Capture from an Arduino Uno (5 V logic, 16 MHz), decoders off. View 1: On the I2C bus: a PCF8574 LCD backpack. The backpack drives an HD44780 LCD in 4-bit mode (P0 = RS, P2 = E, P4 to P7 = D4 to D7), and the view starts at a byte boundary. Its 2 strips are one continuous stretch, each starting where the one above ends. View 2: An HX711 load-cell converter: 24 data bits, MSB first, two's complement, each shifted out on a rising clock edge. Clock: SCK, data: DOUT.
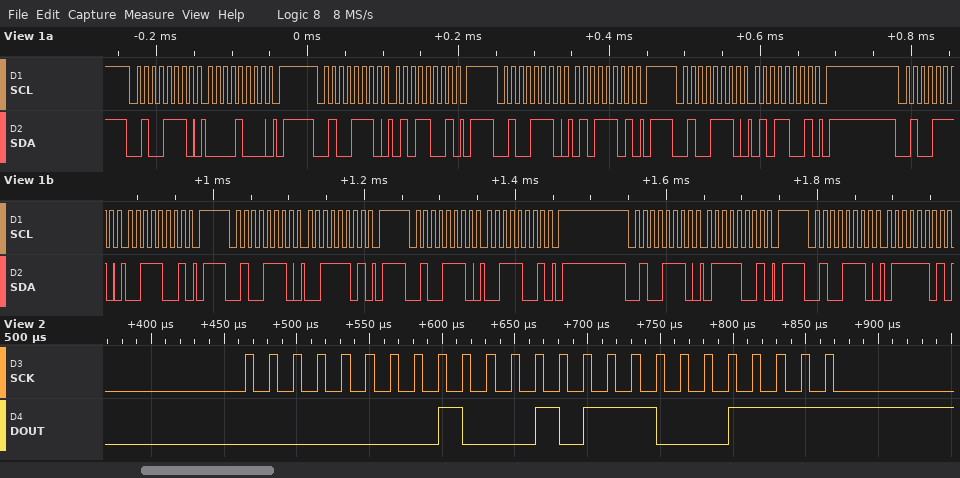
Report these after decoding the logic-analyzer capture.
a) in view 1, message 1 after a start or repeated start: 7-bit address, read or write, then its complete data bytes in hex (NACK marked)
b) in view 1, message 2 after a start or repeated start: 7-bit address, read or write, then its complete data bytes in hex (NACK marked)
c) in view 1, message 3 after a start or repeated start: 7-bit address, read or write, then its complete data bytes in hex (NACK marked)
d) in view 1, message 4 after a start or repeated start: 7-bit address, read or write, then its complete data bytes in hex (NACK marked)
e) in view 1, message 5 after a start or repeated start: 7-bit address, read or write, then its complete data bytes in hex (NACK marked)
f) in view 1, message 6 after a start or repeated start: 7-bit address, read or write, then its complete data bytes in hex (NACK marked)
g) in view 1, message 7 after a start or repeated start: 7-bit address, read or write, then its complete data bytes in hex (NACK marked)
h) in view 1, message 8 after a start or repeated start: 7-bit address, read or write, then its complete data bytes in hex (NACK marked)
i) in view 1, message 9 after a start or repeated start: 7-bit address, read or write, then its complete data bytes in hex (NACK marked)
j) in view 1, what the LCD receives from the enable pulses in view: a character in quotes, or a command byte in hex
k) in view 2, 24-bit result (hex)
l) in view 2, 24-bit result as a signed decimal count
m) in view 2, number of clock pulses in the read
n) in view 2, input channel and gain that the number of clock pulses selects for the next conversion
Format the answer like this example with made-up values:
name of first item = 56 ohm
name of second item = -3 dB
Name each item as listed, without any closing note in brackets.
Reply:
in view 1, message 1 after a start or repeated start: 7-bit address, read or write, then its complete data bytes in hex = 0x27 write: 08
in view 1, message 2 after a start or repeated start: 7-bit address, read or write, then its complete data bytes in hex = 0x27 write: 59
in view 1, message 3 after a start or repeated start: 7-bit address, read or write, then its complete data bytes in hex = 0x27 write: 5D
in view 1, message 4 after a start or repeated start: 7-bit address, read or write, then its complete data bytes in hex = 0x27 write: 59
in view 1, message 5 after a start or repeated start: 7-bit address, read or write, then its complete data bytes in hex = 0x27 write: 39
in view 1, message 6 after a start or repeated start: 7-bit address, read or write, then its complete data bytes in hex = 0x27 write: 3D
in view 1, message 7 after a start or repeated start: 7-bit address, read or write, then its complete data bytes in hex = 0x27 write: 39
in view 1, message 8 after a start or repeated start: 7-bit address, read or write, then its complete data bytes in hex = 0x27 write: 79
in view 1, message 9 after a start or repeated start: 7-bit address, read or write, then its complete data bytes in hex = 0x27 write: 7D
in view 1, what the LCD receives from the enable pulses in view: a character in quotes, or a command byte in hex = 'S'
in view 2, 24-bit result = 0x008B8F
in view 2, 24-bit result as a signed decimal count = 35727
in view 2, number of clock pulses in the read = 25
in view 2, input channel and gain that the number of clock pulses selects for the next conversion = channel A, gain 128
